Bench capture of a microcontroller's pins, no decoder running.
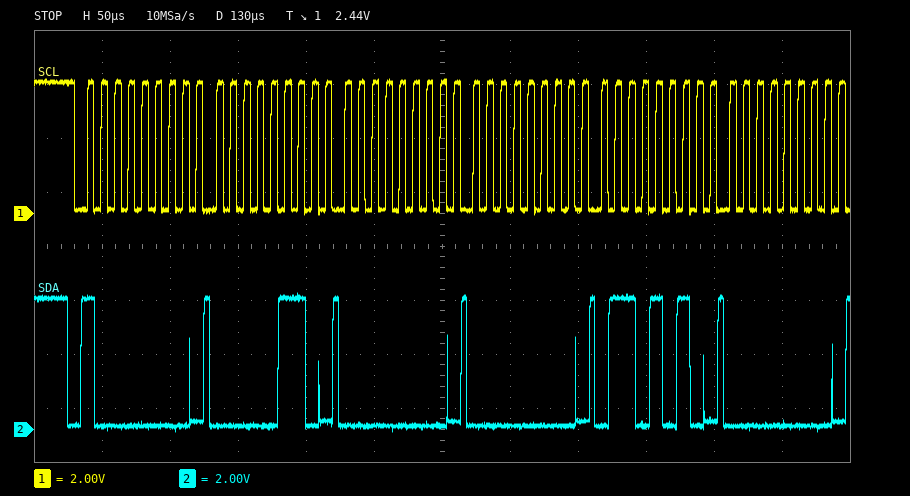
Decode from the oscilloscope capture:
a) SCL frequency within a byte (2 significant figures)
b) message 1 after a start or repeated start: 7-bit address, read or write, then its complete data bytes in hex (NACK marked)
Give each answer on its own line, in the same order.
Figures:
100 kHz
0x40 write: 06 00 00 6A 00
